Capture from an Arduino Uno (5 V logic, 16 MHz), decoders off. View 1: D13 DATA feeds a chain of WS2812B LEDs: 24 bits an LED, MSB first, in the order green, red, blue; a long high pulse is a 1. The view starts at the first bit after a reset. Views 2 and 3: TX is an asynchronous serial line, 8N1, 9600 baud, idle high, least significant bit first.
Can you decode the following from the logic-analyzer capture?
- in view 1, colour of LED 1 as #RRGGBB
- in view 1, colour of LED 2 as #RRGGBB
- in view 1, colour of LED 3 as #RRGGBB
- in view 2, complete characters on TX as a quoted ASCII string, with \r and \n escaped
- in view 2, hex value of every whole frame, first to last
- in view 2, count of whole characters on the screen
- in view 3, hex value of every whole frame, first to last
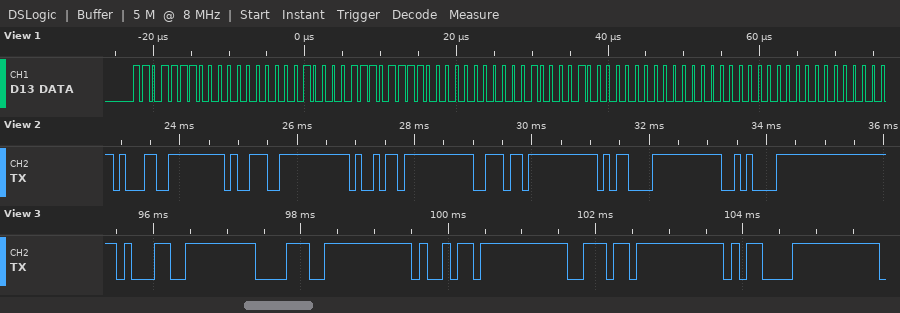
#00DE21
#00DE21
#000000
"19in\r\n"
31 39 69 6E 0D 0A
6
0x31 0x38 0x69 0x6E 0x0D
